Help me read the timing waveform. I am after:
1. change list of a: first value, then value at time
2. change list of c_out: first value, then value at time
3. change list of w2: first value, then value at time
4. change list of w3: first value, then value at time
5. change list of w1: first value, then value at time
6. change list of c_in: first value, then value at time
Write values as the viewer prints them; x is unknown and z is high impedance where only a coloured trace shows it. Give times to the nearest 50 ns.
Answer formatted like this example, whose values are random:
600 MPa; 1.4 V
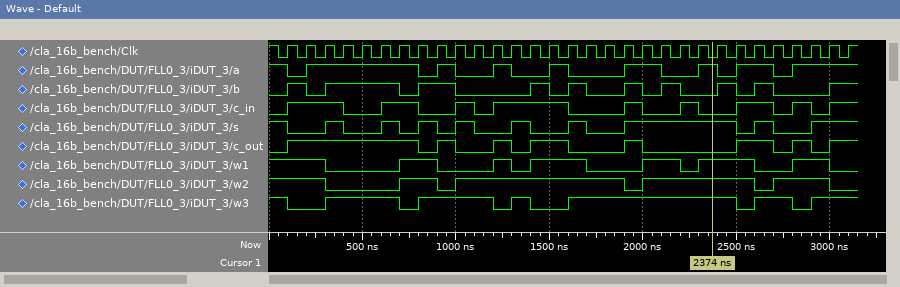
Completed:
1, 0 at 100 ns, 1 at 200 ns, 0 at 800 ns, 1 at 900 ns, 0 at 1000 ns, 1 at 1200 ns, 0 at 1300 ns, 1 at 1500 ns, 0 at 1600 ns, 1 at 1900 ns, 0 at 2100 ns, 1 at 2300 ns, 0 at 2400 ns, 1 at 2500 ns, 0 at 2700 ns, 1 at 2800 ns; 0, 1 at 100 ns, 0 at 800 ns, 1 at 900 ns, 0 at 1000 ns, 1 at 1200 ns, 0 at 1300 ns, 1 at 1400 ns, 0 at 1600 ns, 1 at 1900 ns, 0 at 2000 ns, 1 at 2500 ns, 0 at 2700 ns, 1 at 2800 ns, 0 at 2900 ns, 1 at 3000 ns; 1, 0 at 300 ns, 1 at 700 ns, 0 at 900 ns, 1 at 1000 ns, 0 at 1900 ns, 1 at 2000 ns, 0 at 2600 ns, 1 at 2700 ns, 0 at 3000 ns; 1, 0 at 100 ns, 1 at 300 ns, 0 at 700 ns, 1 at 800 ns, 0 at 1200 ns, 1 at 1300 ns, 0 at 1400 ns, 1 at 1600 ns, 0 at 2500 ns, 1 at 2600 ns, 0 at 2800 ns, 1 at 2900 ns; 1, 0 at 300 ns, 1 at 700 ns, 0 at 900 ns, 1 at 1200 ns, 0 at 1300 ns, 1 at 1400 ns, 0 at 1700 ns, 1 at 2000 ns, 0 at 2200 ns, 1 at 2300 ns, 0 at 2600 ns, 1 at 2800 ns, 0 at 3000 ns; 0, 1 at 100 ns, 0 at 400 ns, 1 at 600 ns, 0 at 800 ns, 1 at 1000 ns, 0 at 1100 ns, 1 at 1200 ns, 0 at 1600 ns, 1 at 1900 ns, 0 at 2000 ns, 1 at 2200 ns, 0 at 2300 ns, 1 at 2500 ns, 0 at 2700 ns, 1 at 2800 ns, 0 at 2900 ns, 1 at 3000 ns
